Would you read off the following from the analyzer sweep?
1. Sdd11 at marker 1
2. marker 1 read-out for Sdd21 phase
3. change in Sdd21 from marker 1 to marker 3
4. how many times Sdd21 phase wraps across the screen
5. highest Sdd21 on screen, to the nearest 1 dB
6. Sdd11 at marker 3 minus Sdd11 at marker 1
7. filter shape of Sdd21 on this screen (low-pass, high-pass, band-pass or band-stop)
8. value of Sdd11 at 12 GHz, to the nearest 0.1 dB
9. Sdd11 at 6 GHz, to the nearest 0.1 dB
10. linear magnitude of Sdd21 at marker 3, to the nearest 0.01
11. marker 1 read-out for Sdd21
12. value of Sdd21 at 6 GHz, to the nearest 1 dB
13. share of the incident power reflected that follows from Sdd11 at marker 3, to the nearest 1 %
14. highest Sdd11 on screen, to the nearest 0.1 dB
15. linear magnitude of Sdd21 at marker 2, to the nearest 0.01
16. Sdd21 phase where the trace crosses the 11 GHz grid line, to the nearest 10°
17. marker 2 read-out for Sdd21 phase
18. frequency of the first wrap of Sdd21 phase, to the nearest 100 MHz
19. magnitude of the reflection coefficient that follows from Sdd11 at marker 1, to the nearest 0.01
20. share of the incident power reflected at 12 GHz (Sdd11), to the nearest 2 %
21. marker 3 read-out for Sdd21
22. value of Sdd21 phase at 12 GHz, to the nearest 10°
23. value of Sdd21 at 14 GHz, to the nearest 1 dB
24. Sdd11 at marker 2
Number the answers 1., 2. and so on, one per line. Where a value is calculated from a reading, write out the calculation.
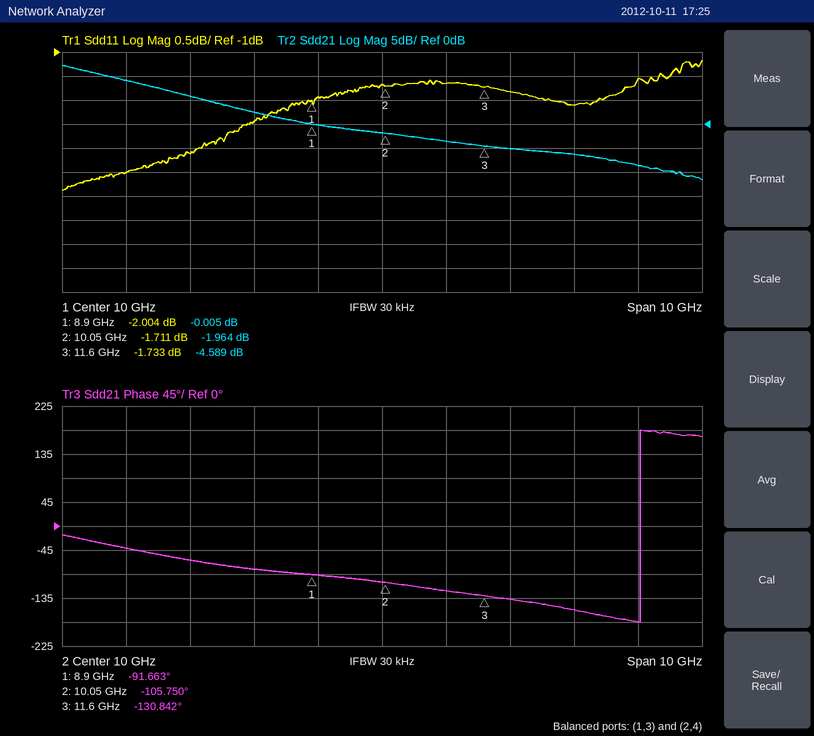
1. -2.004 dB
2. -91.663°
3. -4.589 − (-0.005) = -4.584 dB
4. 1
5. 12 dB
6. -1.733 − (-2.004) = 0.271 dB
7. low-pass
8. -1.8 dB
9. -3.5 dB
10. 10^(-4.589/20) ≈ 0.59
11. -0.005 dB
12. 9 dB
13. 10^(-1.733/10) ≈ 67 %
14. -1.2 dB
15. 10^(-1.964/20) ≈ 0.80
16. -120°
17. -105.750°
18. 14.0 GHz
19. 10^(-2.004/20) ≈ 0.79
20. 10^(-1.8/10) ≈ 66 %
21. -4.589 dB
22. -140°
23. -9 dB
24. -1.711 dB
